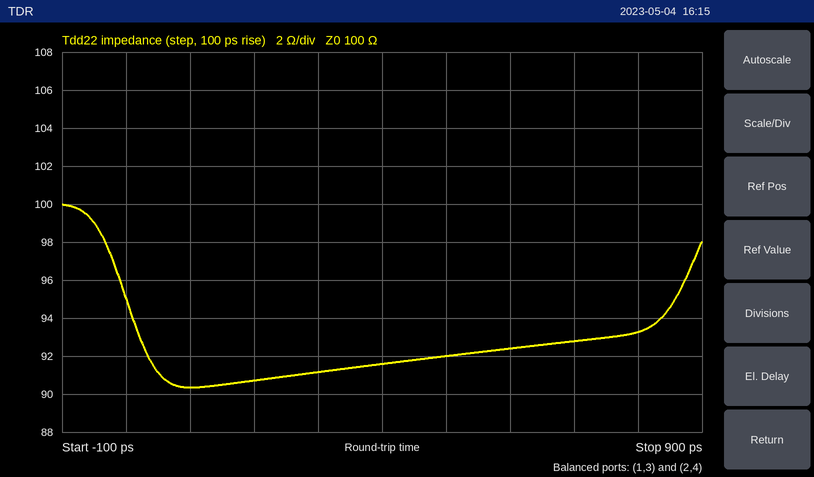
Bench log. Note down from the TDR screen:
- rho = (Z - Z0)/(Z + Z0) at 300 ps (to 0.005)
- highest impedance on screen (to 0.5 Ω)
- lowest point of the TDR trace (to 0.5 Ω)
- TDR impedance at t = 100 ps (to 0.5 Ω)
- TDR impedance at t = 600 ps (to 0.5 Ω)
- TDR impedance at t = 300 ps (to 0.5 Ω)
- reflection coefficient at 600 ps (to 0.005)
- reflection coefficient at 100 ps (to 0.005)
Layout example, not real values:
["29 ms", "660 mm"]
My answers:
["-0.045", "100.0 Ω", "90.5 Ω", "90.5 Ω", "92.5 Ω", "91.0 Ω", "-0.040", "-0.050"]
